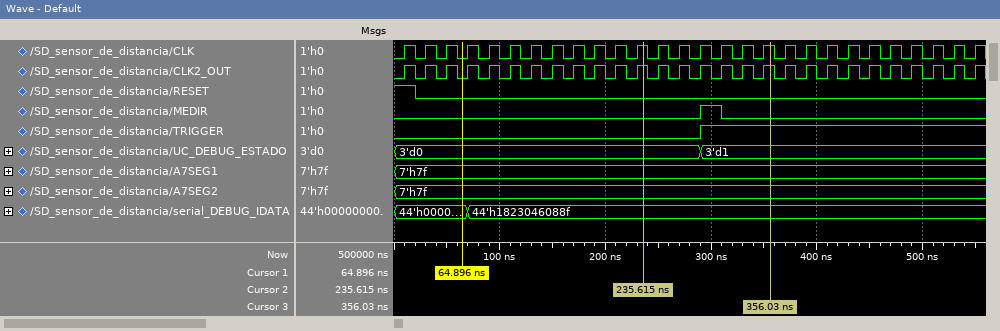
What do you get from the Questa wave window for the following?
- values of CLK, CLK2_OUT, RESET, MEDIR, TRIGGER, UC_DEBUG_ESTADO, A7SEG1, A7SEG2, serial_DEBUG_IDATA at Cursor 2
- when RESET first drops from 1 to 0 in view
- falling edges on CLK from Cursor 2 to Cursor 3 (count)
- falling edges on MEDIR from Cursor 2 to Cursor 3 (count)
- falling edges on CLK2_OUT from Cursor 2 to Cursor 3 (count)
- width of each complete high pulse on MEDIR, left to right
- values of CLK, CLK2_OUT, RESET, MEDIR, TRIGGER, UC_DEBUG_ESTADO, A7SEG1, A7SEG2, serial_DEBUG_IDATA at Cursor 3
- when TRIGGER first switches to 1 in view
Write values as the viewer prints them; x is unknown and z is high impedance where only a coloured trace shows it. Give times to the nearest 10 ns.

CLK=1, CLK2_OUT=1, RESET=0, MEDIR=0, TRIGGER=0, UC_DEBUG_ESTADO=3'd0, A7SEG1=7'h7f, A7SEG2=7'h7f, serial_DEBUG_IDATA=44'h1823046088f
20 ns
6
1
6
20 ns
CLK=1, CLK2_OUT=1, RESET=0, MEDIR=0, TRIGGER=1, UC_DEBUG_ESTADO=3'd1, A7SEG1=7'h7f, A7SEG2=7'h7f, serial_DEBUG_IDATA=44'h1823046088f
290 ns
